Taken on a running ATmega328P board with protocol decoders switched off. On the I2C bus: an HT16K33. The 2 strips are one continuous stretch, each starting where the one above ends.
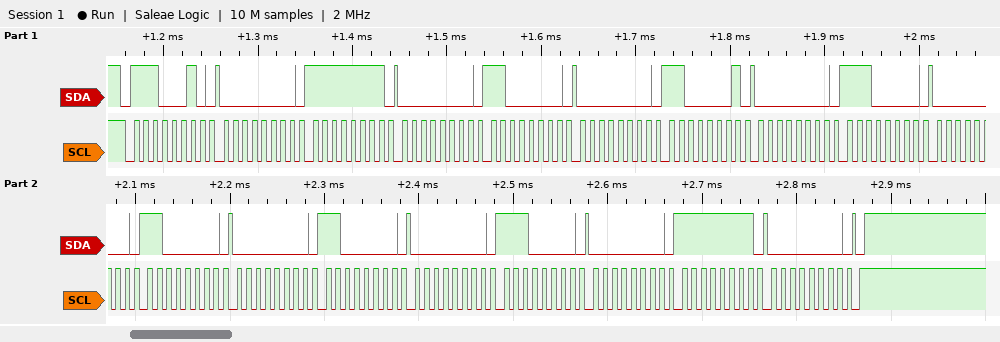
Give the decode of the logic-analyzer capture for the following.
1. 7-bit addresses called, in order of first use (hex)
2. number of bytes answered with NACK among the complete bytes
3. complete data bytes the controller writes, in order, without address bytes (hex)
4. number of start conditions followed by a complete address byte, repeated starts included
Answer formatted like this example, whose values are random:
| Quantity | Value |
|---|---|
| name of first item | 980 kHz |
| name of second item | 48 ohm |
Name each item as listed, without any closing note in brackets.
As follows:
| Quantity | Value |
|---|---|
| 7-bit addresses called, in order of first use | 0x71 |
| number of bytes answered with NACK among the complete bytes | 0 |
| complete data bytes the controller writes, in order, without address bytes | 00 FF 00 C0 00 C1 00 E0 00 C0 00 C0 00 E0 00 FF 00 |
| number of start conditions followed by a complete address byte, repeated starts included | 1 |
